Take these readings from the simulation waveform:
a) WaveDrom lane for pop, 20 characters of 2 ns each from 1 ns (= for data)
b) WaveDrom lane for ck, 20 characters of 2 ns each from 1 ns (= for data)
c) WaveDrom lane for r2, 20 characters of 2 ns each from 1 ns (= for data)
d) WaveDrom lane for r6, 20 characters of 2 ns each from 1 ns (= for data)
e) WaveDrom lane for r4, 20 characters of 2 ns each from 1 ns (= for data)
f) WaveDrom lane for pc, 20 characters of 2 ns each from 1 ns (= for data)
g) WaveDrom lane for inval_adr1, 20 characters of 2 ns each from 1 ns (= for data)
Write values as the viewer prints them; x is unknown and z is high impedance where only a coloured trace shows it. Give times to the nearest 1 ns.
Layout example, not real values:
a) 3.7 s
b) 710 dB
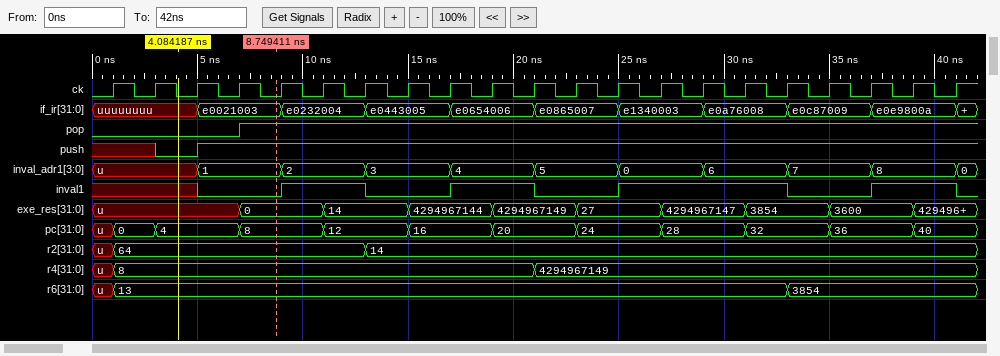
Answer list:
a) {name: 'pop', wave: '0..1................'}
b) {name: 'ck', wave: 'p...................'}
c) {name: 'r2', wave: '=.....=.............', data: '64 14'}
d) {name: 'r6', wave: '=...............=...', data: '13 3854'}
e) {name: 'r4', wave: '=.........=.........', data: '8 4294967149'}
f) {name: 'pc', wave: '==.=.=.=.=.=.=.=.=.=', data: '0 4 8 12 16 20 24 28 32 36 40'}
g) {name: 'inval_adr1', wave: 'x.=.=.=.=.=.=.=.=.=.', data: '1 2 3 4 5 0 6 7 8'}
